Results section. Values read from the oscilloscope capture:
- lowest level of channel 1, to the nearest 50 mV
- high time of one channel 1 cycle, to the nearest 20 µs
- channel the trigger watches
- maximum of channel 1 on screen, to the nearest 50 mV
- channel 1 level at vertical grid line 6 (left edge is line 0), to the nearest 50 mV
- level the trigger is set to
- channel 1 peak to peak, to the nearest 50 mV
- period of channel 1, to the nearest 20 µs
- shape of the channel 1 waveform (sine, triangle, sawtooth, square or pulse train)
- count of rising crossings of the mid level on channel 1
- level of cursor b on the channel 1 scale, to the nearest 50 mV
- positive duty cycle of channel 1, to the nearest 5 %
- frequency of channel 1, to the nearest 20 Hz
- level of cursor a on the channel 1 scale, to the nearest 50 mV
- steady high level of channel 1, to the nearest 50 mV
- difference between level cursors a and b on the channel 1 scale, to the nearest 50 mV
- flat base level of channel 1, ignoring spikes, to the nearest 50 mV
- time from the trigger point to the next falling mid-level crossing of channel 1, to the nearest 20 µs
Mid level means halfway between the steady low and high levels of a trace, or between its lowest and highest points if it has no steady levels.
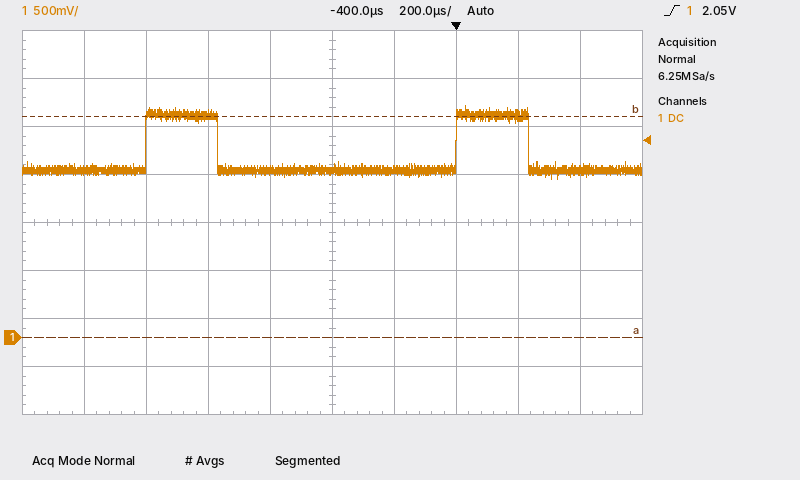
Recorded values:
1.65 V
240 µs
channel 1
2.40 V
1.75 V
2.05 V
750 mV
1.00 ms
pulse train
2
2.30 V
25 %
1.00 kHz
0 mV
2.30 V
2.30 V
1.75 V
240 µs
